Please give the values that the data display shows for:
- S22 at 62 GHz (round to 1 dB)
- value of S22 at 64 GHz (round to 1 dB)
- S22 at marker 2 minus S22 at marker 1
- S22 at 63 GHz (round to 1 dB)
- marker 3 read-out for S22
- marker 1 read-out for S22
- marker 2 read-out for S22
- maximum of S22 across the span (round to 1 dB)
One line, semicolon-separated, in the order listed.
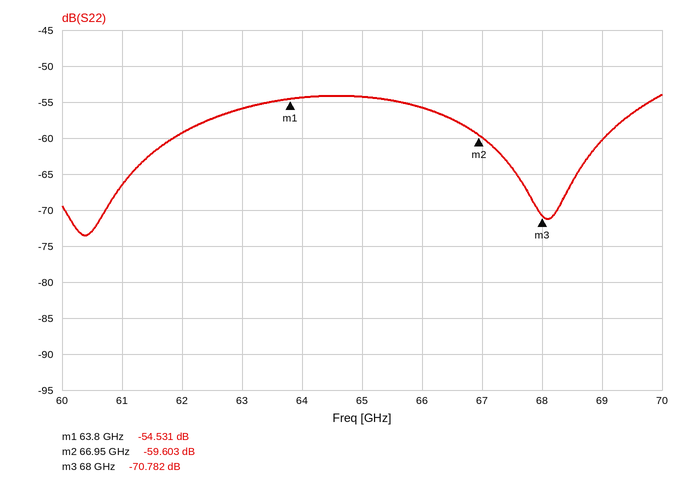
-59 dB; -54 dB; -5.072 dB; -56 dB; -70.782 dB; -54.531 dB; -59.603 dB; -54 dB
